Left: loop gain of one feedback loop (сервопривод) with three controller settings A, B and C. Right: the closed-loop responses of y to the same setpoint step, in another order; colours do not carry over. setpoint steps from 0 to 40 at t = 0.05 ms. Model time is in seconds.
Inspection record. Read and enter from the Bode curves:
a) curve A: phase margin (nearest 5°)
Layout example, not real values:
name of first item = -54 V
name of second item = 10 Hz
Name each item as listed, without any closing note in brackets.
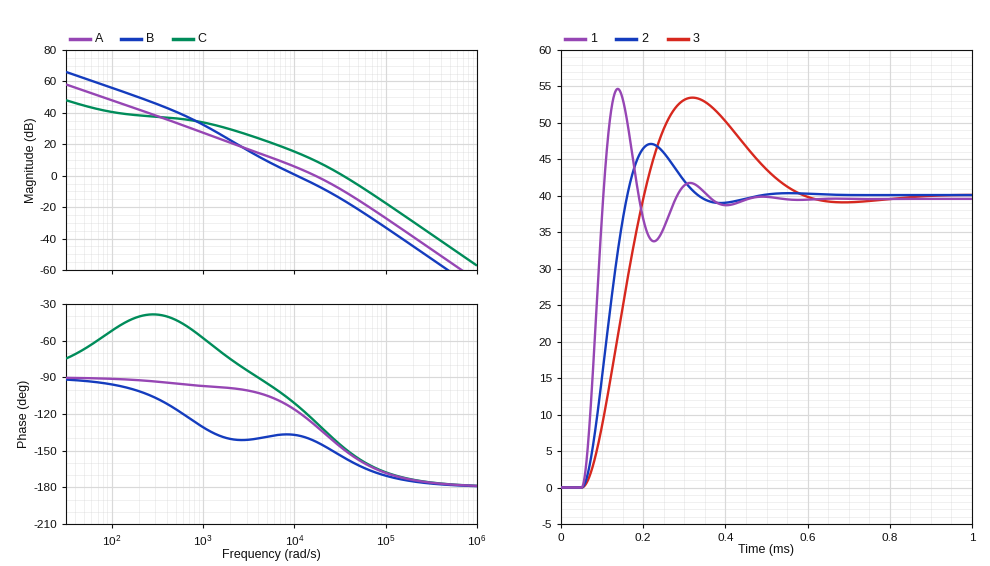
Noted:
curve A: phase margin = 50°
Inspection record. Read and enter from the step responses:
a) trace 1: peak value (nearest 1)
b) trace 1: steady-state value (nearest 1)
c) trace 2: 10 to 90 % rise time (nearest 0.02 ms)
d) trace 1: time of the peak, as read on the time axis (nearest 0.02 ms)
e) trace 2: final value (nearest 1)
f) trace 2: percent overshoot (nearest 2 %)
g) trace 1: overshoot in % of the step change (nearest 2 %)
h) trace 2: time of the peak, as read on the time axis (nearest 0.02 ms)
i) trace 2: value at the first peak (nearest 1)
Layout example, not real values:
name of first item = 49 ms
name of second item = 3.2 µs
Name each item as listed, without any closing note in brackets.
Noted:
trace 1: peak value = 55
trace 1: steady-state value = 40
trace 2: 10 to 90 % rise time = 0.08 ms
trace 1: time of the peak, as read on the time axis = 0.14 ms
trace 2: final value = 40
trace 2: percent overshoot = 18 %
trace 1: overshoot in % of the step change = 38 %
trace 2: time of the peak, as read on the time axis = 0.22 ms
trace 2: value at the first peak = 47
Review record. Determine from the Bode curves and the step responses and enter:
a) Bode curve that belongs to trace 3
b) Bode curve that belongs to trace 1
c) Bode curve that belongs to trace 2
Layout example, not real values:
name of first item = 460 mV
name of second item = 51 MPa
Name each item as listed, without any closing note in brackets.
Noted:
Bode curve that belongs to trace 3 = B
Bode curve that belongs to trace 1 = C
Bode curve that belongs to trace 2 = A
